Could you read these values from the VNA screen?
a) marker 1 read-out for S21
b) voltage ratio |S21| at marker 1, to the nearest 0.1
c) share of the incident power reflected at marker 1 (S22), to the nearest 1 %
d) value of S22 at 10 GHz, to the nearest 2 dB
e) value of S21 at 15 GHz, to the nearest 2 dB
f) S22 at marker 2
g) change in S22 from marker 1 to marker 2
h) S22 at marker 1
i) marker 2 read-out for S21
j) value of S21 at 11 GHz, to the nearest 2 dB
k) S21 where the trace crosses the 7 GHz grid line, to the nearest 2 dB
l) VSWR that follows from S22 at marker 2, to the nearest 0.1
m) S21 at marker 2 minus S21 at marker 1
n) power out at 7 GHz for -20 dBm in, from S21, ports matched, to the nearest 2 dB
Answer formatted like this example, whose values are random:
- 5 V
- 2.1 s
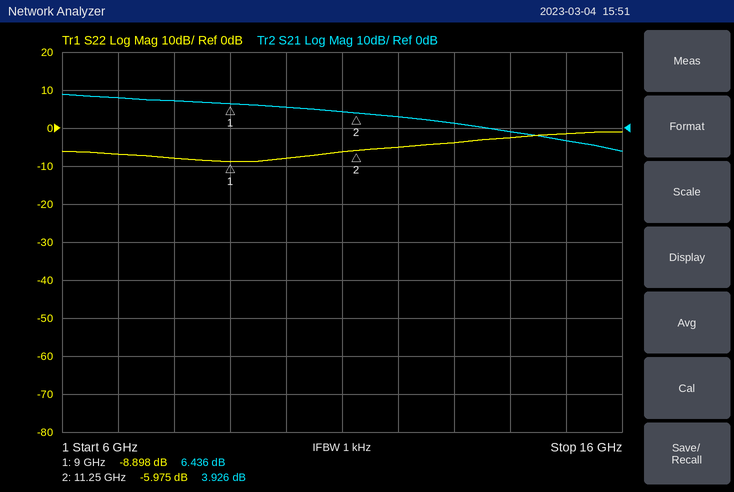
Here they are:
- 6.436 dB
- 2.1
- 13 %
- -8 dB
- -4 dB
- -5.975 dB
- 2.923 dB
- -8.898 dB
- 3.926 dB
- 4 dB
- 8 dB
- 3.0
- -2.510 dB
- -12 dBm
